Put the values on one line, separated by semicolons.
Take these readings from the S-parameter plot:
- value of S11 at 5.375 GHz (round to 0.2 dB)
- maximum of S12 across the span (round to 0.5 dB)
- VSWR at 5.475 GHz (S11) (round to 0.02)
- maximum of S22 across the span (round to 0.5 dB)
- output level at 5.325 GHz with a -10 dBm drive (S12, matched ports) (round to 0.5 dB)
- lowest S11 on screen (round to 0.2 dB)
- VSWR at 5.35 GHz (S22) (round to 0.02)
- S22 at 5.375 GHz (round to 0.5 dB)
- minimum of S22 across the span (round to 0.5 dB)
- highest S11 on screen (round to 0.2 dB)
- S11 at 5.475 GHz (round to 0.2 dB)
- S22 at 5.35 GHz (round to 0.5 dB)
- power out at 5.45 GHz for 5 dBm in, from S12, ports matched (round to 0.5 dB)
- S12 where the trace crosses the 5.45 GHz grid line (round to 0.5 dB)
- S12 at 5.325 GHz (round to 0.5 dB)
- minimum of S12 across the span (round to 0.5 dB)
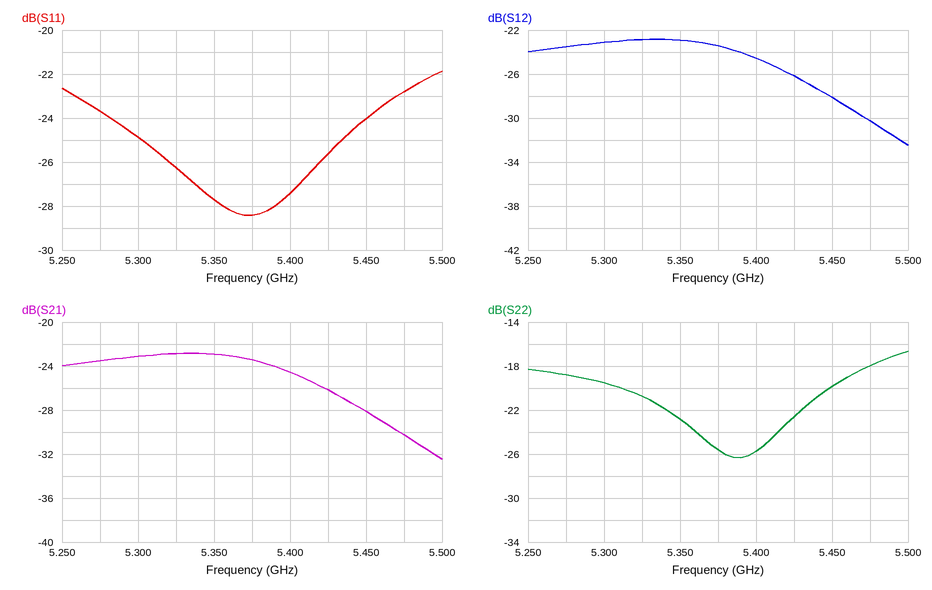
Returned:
-28.4 dB; -23.0 dB; 1.16; -16.5 dB; -33.0 dBm; -28.4 dB; 1.16; -25.5 dB; -26.5 dB; -21.8 dB; -22.8 dB; -23.0 dB; -23.0 dBm; -28.0 dB; -23.0 dB; -32.5 dB
